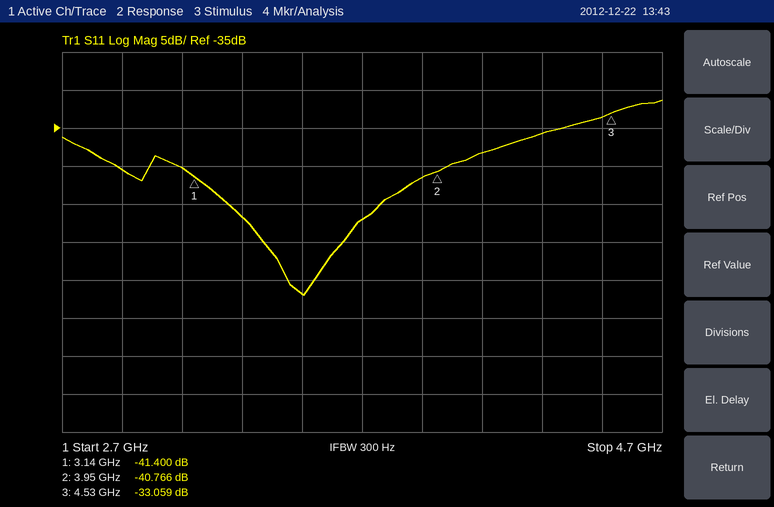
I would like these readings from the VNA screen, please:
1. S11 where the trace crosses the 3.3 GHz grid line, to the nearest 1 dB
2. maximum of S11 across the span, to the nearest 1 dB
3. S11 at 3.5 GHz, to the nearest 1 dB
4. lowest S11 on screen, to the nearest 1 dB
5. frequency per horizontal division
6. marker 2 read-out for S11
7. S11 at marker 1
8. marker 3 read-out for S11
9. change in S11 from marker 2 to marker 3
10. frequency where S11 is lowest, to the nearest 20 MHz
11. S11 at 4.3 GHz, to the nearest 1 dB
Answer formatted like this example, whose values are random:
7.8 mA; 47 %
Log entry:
-47 dB; -31 dB; -57 dB; -57 dB; 200 MHz; -40.766 dB; -41.400 dB; -33.059 dB; 7.707 dB; 3.50 GHz; -36 dB
